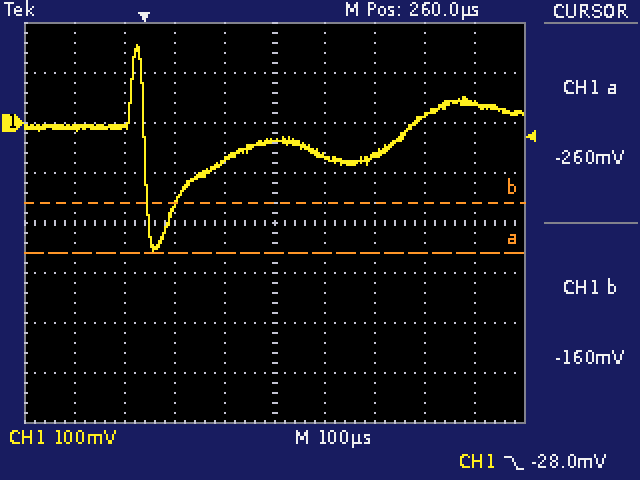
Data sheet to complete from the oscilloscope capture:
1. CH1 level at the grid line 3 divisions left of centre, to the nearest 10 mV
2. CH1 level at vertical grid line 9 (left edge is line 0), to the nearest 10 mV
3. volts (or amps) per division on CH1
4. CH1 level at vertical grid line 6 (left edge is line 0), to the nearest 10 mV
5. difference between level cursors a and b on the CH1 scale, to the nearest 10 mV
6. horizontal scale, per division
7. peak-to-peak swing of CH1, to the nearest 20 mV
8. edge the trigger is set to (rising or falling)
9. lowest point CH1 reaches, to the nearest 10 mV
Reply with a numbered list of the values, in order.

1. -10 mV
2. 40 mV
3. 100 mV
4. -70 mV
5. 100 mV
6. 100 µs
7. 420 mV
8. falling
9. -260 mV
